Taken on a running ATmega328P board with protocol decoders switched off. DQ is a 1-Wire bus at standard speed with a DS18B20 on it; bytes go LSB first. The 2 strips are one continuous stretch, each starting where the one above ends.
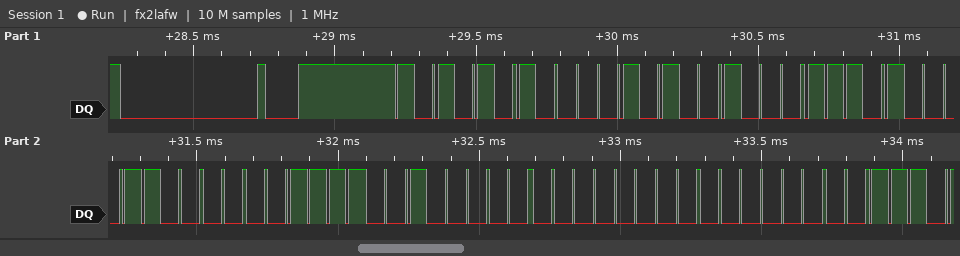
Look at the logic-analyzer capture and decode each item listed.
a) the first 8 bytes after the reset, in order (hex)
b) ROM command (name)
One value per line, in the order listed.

55 28 71 31 F0 04 00 00
Match ROM
